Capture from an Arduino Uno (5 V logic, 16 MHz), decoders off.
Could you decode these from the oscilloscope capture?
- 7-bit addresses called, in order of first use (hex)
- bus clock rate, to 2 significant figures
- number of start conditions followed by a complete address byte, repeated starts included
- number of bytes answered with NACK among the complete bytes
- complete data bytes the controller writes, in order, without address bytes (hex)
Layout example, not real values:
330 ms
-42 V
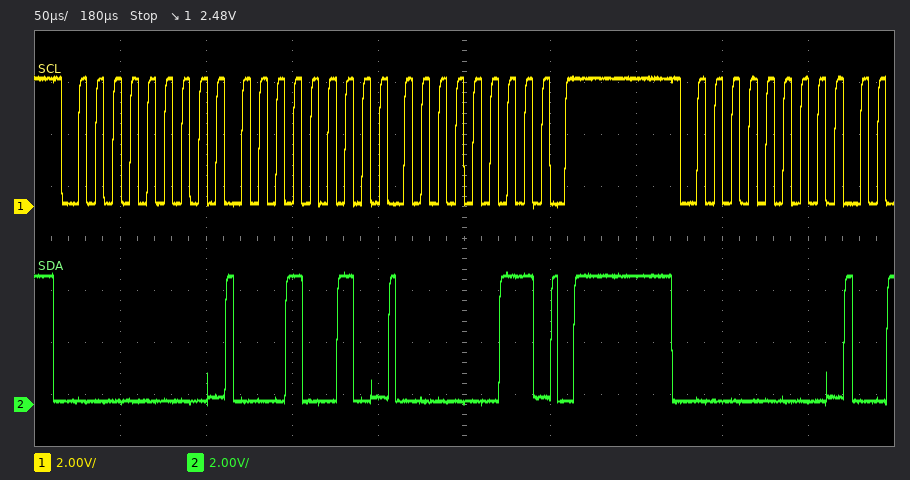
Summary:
0x00
100 kHz
2
0
12 03
